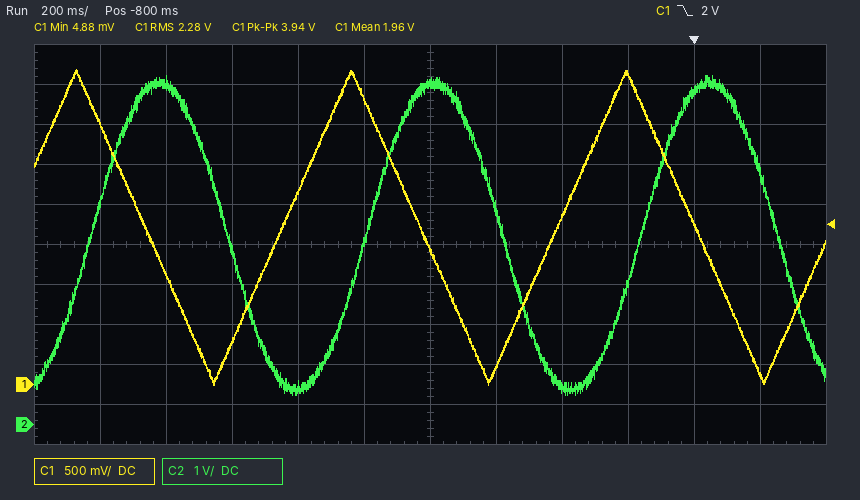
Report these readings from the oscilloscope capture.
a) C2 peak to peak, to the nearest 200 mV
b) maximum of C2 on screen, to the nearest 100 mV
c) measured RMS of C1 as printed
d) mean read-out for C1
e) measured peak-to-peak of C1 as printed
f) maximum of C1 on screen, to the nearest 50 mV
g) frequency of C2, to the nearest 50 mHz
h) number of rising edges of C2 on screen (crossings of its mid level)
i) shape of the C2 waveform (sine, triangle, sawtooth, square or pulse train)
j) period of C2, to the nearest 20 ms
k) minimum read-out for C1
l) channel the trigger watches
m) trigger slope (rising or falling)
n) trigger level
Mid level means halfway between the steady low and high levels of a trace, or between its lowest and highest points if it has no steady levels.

8.0 V
8.7 V
2.28 V
1.96 V
3.94 V
3.95 V
1.20 Hz
3
sine
840 ms
4.88 mV
C1
falling
2 V
